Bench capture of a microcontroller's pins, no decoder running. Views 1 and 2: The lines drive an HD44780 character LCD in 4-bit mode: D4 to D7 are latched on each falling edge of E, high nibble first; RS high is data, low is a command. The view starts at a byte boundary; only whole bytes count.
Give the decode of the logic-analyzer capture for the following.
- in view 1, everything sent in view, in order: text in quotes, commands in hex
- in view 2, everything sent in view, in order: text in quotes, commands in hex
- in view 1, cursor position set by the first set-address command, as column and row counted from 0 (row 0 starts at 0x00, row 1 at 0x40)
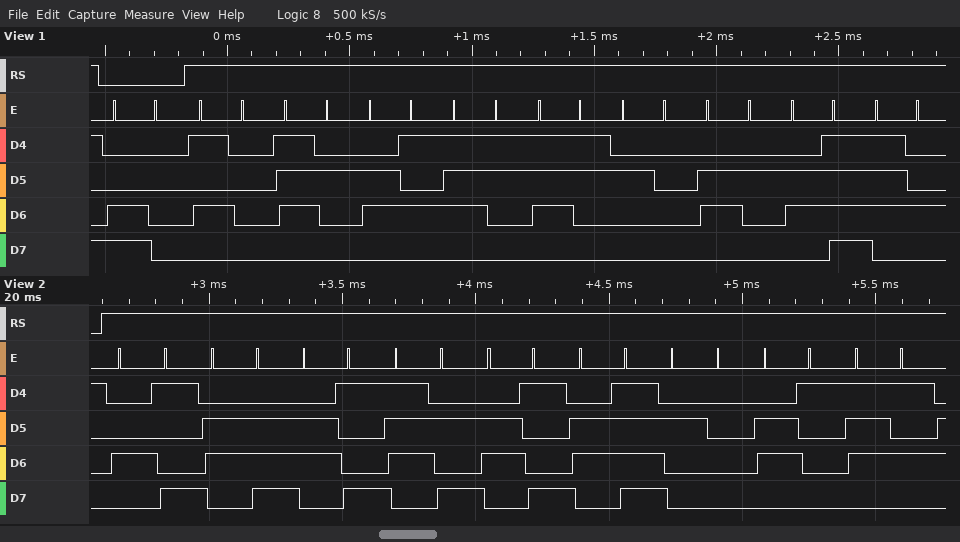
0xC0 "Press bot"
"Inizio au"
column 0, row 1
